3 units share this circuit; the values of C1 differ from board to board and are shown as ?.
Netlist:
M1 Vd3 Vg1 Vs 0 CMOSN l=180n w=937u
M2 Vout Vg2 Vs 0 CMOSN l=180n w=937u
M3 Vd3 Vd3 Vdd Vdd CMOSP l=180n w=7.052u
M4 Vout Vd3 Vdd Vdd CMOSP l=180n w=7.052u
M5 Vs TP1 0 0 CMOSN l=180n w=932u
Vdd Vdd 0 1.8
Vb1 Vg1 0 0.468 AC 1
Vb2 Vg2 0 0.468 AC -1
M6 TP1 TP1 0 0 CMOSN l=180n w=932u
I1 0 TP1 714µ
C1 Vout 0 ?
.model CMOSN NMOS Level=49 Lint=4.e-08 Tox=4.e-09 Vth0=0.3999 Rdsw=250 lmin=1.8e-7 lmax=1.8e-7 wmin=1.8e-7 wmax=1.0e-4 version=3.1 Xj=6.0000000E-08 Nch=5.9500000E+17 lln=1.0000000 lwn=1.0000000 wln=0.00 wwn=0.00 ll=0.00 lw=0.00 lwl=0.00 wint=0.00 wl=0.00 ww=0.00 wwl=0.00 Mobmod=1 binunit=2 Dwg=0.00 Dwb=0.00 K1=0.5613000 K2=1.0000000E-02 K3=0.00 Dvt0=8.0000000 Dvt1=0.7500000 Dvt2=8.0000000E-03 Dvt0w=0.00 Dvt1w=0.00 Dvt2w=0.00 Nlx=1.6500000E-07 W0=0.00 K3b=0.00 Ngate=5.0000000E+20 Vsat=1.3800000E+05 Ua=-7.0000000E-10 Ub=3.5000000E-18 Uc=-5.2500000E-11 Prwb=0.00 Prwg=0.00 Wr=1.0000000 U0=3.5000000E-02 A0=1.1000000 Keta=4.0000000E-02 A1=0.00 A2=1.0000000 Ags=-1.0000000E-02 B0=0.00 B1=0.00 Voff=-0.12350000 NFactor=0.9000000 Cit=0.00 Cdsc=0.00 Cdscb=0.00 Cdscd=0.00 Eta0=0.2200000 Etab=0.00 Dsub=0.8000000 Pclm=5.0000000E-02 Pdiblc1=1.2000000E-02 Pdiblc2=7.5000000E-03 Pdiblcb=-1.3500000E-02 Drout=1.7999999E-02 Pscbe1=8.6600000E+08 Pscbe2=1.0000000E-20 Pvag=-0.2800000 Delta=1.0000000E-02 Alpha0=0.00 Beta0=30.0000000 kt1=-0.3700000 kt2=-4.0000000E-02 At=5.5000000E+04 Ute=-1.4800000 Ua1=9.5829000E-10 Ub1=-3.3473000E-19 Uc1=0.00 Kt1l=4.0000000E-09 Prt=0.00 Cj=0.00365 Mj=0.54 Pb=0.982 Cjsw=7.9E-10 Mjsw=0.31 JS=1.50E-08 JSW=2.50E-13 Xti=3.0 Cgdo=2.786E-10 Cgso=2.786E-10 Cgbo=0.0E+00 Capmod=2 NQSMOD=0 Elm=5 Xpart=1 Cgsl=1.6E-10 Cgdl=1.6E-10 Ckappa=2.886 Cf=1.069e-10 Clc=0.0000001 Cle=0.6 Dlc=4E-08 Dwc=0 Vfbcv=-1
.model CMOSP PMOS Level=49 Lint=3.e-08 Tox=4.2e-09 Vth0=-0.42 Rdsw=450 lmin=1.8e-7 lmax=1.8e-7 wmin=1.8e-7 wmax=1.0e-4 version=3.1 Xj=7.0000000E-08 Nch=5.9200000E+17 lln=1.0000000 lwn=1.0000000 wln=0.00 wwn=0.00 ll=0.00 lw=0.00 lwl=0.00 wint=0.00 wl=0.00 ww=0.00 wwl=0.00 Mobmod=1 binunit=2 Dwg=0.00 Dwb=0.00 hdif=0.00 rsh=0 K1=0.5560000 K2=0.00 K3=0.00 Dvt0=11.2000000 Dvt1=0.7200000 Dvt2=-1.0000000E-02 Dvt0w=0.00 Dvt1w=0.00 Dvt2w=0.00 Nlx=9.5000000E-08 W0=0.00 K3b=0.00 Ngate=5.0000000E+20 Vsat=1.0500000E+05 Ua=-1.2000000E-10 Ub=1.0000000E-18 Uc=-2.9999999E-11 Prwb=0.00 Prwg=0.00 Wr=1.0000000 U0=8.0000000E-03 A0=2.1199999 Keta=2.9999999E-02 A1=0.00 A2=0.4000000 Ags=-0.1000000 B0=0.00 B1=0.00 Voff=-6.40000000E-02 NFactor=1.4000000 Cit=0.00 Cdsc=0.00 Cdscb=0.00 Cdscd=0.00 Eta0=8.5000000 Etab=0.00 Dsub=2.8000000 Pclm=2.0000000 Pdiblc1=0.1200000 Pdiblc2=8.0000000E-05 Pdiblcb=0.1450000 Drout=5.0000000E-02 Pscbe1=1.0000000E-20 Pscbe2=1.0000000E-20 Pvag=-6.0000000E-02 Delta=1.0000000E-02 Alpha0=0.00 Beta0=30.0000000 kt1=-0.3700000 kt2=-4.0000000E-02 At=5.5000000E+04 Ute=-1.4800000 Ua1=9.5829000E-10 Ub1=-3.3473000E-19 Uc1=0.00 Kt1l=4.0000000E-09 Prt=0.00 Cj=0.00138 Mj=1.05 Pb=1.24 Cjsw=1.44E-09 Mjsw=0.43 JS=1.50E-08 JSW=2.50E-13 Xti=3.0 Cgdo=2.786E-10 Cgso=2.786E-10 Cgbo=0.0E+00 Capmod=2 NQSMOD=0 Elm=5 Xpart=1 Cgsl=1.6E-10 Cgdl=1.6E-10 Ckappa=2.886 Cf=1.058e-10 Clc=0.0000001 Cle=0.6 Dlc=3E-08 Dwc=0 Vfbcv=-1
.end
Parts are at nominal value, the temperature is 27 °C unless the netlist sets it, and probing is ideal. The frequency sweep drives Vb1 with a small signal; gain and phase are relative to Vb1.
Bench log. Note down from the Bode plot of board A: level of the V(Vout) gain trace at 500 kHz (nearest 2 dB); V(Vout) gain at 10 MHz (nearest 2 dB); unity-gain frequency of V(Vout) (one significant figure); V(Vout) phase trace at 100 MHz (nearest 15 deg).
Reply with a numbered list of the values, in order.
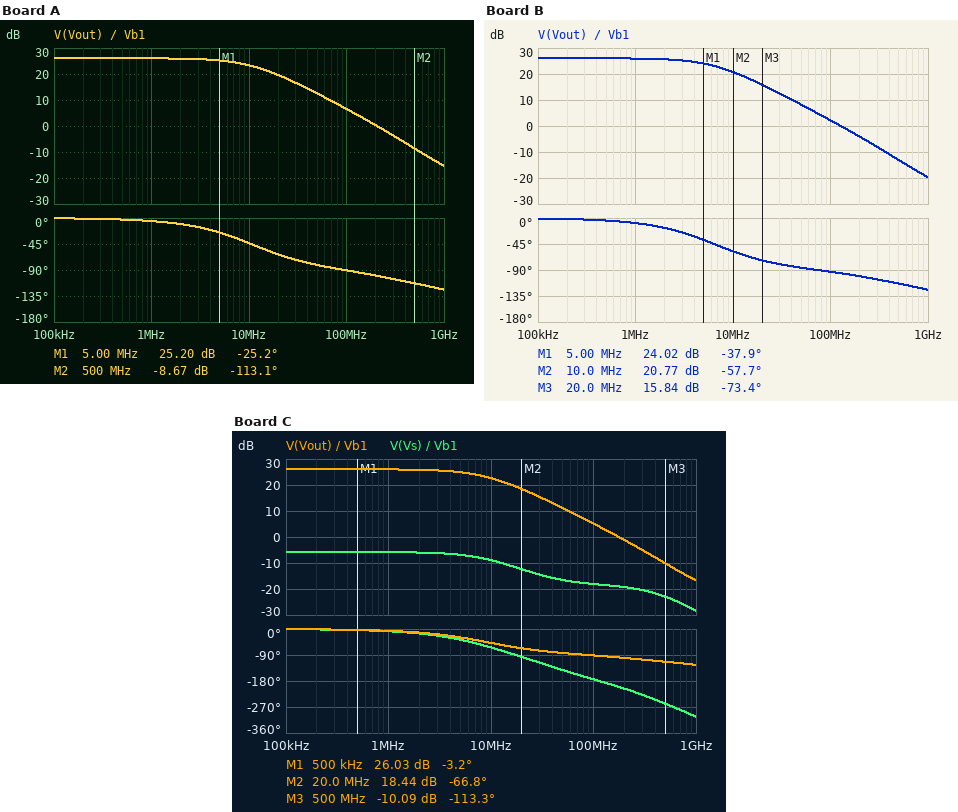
1. 26 dB
2. 24 dB
3. 200 MHz
4. -90 deg
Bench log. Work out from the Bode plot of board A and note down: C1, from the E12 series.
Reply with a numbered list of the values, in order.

1. 6.8 pF
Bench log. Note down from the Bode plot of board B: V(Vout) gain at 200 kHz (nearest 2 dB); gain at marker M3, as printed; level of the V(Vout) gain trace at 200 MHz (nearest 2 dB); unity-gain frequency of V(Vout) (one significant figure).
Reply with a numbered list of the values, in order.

1. 26 dB
2. 15.84 dB
3. -4 dB
4. 100 MHz
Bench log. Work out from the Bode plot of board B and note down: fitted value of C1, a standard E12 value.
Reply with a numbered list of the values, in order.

1. 12 pF
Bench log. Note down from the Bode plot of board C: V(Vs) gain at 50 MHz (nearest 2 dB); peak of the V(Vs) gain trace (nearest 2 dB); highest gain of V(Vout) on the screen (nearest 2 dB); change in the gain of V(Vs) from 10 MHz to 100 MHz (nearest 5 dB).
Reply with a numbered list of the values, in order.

1. -16 dB
2. -6 dB
3. 26 dB
4. -10 dB
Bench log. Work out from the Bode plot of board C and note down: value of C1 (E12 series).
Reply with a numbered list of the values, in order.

1. 8.2 pF
